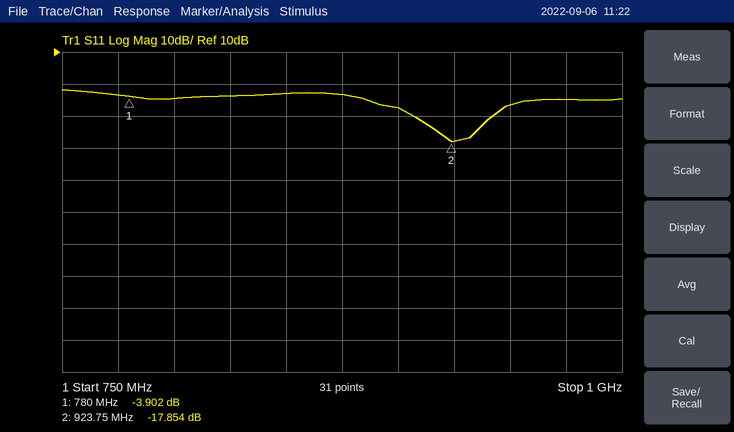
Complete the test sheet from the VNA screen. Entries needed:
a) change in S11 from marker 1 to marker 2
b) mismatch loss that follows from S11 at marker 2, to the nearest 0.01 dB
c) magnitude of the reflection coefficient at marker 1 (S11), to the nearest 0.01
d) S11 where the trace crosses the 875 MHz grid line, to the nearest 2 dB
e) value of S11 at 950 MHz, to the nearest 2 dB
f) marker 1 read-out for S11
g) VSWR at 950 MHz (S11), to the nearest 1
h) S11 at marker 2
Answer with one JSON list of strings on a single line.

["-13.952 dB", "0.07 dB", "0.64", "-4 dB", "-6 dB", "-3.902 dB", "3", "-17.854 dB"]
